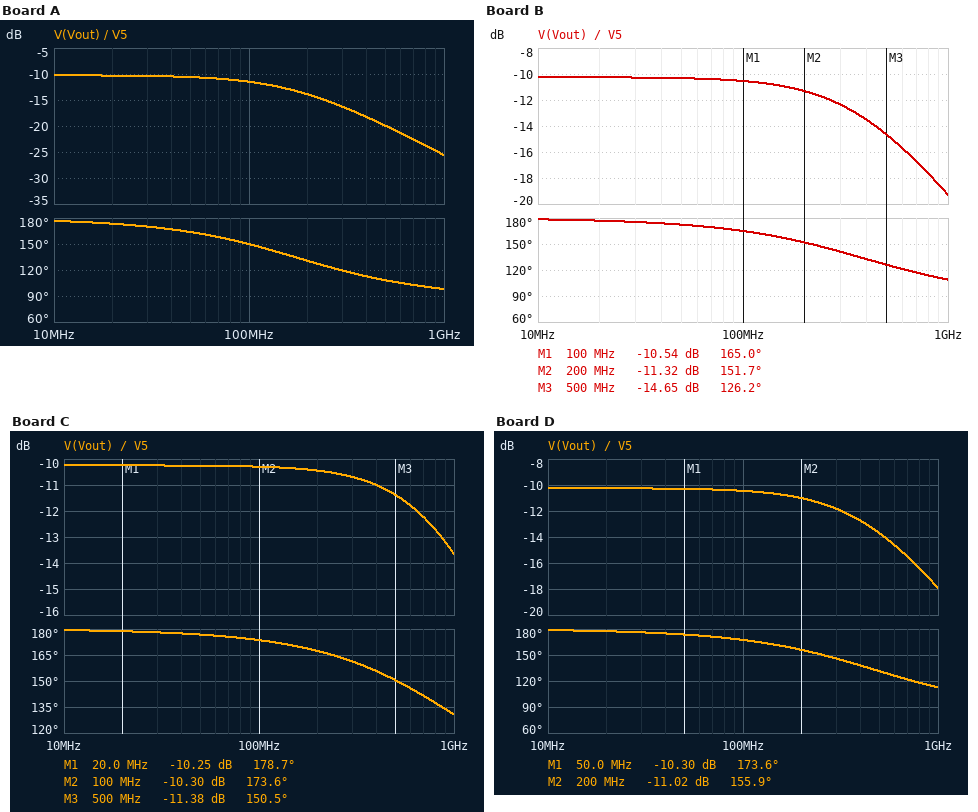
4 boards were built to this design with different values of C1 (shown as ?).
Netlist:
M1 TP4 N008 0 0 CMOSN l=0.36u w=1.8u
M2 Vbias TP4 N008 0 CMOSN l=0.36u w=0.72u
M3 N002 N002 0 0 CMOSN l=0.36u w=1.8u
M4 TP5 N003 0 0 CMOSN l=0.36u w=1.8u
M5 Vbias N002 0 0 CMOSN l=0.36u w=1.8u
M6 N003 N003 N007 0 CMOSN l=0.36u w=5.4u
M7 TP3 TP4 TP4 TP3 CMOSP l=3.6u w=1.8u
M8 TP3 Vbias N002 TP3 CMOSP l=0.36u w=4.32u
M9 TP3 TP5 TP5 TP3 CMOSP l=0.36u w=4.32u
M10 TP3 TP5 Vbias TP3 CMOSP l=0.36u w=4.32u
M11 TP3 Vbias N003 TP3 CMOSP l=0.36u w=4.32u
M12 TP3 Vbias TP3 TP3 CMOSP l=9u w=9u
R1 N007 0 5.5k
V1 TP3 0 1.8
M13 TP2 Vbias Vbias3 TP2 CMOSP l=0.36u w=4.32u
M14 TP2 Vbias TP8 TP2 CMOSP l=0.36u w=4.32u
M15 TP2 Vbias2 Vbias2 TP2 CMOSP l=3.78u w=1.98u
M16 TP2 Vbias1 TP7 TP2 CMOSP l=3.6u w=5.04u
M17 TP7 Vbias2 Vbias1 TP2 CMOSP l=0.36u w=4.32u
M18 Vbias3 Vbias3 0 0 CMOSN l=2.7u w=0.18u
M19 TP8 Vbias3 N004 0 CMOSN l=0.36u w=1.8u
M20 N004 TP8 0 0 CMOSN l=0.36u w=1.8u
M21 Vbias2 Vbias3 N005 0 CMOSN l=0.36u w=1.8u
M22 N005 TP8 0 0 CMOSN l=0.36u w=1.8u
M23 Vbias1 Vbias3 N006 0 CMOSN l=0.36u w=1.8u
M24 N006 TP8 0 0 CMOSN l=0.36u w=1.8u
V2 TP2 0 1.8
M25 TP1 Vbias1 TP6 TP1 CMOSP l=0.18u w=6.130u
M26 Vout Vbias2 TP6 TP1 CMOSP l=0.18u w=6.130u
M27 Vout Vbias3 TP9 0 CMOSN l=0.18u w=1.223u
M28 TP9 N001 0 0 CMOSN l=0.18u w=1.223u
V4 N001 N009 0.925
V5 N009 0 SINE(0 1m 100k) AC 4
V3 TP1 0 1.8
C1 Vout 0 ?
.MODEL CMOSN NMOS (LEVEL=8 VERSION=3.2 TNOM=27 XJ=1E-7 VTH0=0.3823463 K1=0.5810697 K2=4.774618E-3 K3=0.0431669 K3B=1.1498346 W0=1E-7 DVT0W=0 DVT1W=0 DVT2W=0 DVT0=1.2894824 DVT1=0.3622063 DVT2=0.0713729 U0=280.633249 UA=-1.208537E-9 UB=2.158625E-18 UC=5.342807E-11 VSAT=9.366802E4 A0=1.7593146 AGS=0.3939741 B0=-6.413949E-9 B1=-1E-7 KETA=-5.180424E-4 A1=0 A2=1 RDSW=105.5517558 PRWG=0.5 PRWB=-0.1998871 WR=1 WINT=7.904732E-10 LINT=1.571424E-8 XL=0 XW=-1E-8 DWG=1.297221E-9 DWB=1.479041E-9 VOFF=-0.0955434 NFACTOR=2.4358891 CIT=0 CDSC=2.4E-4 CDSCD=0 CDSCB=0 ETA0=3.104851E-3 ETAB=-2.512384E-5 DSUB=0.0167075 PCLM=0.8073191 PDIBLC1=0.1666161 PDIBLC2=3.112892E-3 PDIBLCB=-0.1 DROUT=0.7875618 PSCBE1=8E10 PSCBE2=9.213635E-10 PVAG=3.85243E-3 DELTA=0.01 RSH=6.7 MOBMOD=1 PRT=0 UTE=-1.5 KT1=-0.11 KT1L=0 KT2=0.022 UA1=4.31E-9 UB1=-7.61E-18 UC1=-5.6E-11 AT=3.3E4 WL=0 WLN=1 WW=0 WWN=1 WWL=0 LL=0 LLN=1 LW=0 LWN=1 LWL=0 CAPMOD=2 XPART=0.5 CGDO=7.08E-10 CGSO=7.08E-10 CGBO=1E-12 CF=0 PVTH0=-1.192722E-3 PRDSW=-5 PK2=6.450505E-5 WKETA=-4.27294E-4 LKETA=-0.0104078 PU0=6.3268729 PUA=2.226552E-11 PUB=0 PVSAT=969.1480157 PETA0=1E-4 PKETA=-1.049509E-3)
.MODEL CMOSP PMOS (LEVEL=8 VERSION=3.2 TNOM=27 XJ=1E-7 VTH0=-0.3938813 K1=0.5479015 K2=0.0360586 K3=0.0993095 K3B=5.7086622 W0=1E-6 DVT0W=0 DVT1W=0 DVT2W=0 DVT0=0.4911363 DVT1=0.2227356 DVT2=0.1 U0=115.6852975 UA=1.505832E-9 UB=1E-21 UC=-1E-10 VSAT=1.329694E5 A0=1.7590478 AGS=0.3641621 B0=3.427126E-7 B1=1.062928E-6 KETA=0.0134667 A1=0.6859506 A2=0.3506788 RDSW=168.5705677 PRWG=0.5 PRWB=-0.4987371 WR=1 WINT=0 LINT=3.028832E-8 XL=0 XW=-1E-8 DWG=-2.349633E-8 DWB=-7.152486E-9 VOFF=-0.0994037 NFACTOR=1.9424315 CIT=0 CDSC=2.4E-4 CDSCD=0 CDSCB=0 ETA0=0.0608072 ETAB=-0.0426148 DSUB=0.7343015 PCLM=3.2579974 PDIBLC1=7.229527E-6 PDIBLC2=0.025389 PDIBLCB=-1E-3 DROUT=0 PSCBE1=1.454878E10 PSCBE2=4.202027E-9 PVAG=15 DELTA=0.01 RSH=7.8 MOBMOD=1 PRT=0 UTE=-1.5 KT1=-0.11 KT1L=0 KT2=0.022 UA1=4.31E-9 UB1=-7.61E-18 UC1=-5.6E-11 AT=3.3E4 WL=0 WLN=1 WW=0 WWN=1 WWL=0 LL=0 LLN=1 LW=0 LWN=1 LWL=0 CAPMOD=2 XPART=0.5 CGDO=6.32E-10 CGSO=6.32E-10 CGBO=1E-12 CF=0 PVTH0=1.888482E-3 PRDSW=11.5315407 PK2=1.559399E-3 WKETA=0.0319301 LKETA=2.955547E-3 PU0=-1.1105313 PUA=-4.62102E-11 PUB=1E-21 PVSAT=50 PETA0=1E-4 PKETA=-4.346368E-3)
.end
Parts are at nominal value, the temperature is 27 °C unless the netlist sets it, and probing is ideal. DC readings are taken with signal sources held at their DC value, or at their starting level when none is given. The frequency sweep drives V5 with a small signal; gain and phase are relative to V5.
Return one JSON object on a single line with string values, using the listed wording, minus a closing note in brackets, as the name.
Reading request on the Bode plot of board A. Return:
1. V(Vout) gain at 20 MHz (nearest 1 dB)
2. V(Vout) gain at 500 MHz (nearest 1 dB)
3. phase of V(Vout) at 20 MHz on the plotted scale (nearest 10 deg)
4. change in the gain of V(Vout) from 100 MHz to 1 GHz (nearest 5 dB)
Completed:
{"V(Vout) gain at 20 MHz": "-10 dB", "V(Vout) gain at 500 MHz": "-20 dB", "phase of V(Vout) at 20 MHz on the plotted scale": "170 deg", "change in the gain of V(Vout) from 100 MHz to 1 GHz": "-15 dB"}
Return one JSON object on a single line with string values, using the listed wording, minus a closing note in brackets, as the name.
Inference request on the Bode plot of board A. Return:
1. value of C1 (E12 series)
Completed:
{"value of C1": "1.8 pF"}
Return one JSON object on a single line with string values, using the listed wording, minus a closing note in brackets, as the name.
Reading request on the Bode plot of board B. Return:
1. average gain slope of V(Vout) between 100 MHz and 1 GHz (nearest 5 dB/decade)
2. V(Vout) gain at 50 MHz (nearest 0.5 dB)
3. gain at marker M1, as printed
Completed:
{"average gain slope of V(Vout) between 100 MHz and 1 GHz": "-10 dB/decade", "V(Vout) gain at 50 MHz": "-10.5 dB", "gain at marker M1, as printed": "-10.54 dB"}
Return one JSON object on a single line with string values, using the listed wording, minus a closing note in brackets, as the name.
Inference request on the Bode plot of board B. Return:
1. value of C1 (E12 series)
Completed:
{"value of C1": "820 fF"}
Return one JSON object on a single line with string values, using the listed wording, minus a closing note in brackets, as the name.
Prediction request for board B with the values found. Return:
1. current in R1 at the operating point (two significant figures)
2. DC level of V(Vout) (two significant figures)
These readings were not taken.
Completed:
{"current in R1 at the operating point": "160 µA", "DC level of V(Vout)": "1.6 V"}
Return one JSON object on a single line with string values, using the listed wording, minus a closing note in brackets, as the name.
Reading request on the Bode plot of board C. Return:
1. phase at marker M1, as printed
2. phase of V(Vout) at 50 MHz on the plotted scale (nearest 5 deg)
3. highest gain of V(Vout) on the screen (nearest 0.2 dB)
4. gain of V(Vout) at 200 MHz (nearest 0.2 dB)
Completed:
{"phase at marker M1, as printed": "178.7 deg", "phase of V(Vout) at 50 MHz on the plotted scale": "175 deg", "highest gain of V(Vout) on the screen": "-10.2 dB", "gain of V(Vout) at 200 MHz": "-10.4 dB"}
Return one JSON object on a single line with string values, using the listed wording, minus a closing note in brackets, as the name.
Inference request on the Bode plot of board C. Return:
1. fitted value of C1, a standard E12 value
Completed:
{"fitted value of C1, a standard E12 value": "330 fF"}
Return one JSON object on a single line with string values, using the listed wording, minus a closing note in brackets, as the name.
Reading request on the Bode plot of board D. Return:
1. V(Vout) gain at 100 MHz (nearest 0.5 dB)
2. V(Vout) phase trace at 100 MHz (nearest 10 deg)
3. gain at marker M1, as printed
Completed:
{"V(Vout) gain at 100 MHz": "-10.5 dB", "V(Vout) phase trace at 100 MHz": "170 deg", "gain at marker M1, as printed": "-10.30 dB"}
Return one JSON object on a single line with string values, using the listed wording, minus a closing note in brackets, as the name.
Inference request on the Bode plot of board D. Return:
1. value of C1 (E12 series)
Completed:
{"value of C1": "680 fF"}
